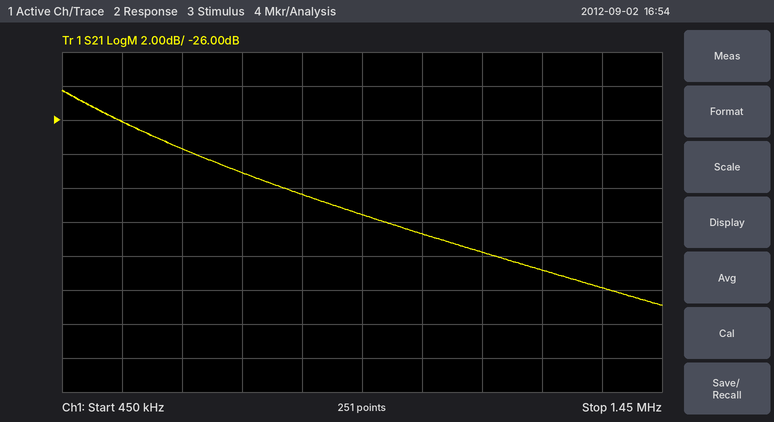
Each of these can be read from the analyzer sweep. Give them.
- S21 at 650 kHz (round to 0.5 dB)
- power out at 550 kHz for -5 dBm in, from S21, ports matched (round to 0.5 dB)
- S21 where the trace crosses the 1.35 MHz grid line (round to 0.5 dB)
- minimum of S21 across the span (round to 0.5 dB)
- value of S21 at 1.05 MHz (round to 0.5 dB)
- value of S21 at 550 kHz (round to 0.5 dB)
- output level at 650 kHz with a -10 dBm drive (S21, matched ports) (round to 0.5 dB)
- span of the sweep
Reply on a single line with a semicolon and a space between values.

-27.5 dB; -31.0 dBm; -36.0 dB; -37.0 dB; -32.5 dB; -26.0 dB; -37.5 dBm; 1 MHz
